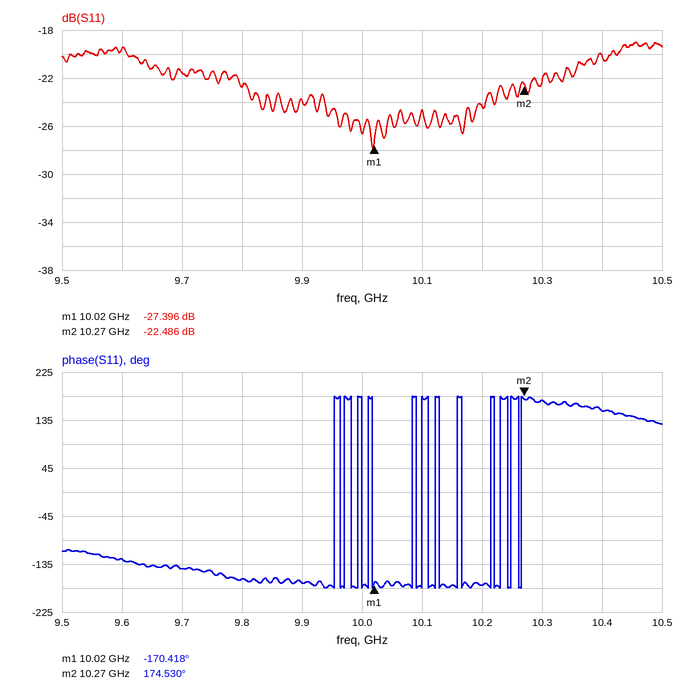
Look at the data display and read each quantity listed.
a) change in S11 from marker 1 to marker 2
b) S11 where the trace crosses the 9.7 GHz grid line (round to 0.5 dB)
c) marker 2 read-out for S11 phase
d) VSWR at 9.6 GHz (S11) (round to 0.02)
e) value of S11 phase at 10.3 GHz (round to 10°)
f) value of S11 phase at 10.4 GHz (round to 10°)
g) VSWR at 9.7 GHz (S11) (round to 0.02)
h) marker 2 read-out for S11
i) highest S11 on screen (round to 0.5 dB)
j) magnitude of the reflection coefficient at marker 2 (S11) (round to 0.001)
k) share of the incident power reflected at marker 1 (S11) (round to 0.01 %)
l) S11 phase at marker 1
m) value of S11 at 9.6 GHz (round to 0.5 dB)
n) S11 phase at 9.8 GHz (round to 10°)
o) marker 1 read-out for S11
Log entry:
4.910 dB
-21.5 dB
174.530°
1.24
170°
150°
1.18
-22.486 dB
-19.0 dB
0.075
0.18 %
-170.418°
-19.5 dB
-160°
-27.396 dB
